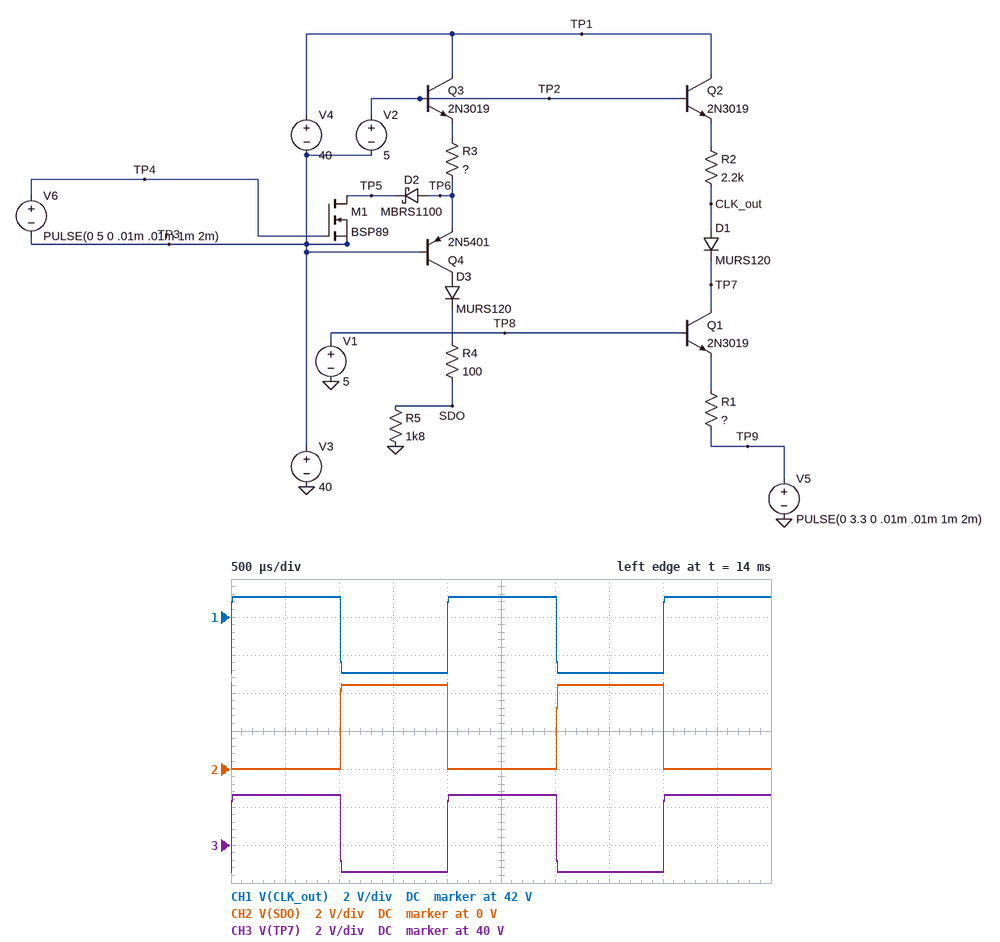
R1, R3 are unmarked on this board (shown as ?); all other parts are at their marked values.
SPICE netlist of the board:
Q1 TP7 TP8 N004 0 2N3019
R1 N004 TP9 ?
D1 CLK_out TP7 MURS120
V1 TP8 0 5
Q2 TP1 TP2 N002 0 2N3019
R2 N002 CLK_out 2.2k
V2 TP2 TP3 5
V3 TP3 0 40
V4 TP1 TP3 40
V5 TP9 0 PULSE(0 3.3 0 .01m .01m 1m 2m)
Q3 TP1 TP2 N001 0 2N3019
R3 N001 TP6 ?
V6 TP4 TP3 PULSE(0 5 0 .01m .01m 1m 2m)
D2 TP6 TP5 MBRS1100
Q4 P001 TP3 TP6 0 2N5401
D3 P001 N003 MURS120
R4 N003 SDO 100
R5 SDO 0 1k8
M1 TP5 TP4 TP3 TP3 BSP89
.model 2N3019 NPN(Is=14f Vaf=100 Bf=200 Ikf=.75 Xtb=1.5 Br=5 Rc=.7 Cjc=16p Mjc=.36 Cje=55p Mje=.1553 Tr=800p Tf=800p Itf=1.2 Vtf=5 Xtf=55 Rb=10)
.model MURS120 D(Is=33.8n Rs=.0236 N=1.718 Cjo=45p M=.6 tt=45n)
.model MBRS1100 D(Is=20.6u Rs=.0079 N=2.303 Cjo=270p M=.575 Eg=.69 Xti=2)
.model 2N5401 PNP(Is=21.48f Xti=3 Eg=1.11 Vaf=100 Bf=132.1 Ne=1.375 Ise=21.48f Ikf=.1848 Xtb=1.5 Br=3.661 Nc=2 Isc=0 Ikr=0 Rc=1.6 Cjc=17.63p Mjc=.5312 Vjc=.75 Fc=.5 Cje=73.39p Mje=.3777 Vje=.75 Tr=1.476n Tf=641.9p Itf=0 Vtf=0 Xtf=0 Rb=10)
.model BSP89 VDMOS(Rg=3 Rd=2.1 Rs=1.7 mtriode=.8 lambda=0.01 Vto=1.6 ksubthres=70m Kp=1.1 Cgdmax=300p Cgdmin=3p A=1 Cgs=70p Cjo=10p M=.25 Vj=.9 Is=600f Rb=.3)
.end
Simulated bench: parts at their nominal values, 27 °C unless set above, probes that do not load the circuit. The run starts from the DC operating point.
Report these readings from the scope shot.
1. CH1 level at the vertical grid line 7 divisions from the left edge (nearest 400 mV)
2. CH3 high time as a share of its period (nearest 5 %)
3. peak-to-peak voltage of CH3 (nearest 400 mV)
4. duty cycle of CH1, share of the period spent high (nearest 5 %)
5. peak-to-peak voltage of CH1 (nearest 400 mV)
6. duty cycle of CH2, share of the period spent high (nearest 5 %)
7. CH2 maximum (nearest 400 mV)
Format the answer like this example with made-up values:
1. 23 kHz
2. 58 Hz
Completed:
1. 39.2 V
2. 50 %
3. 4.0 V
4. 50 %
5. 4.0 V
6. 50 %
7. 4.4 V
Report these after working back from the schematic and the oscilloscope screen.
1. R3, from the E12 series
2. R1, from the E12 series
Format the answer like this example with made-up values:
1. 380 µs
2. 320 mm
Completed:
1. 1.5 kΩ
2. 1.8 kΩ
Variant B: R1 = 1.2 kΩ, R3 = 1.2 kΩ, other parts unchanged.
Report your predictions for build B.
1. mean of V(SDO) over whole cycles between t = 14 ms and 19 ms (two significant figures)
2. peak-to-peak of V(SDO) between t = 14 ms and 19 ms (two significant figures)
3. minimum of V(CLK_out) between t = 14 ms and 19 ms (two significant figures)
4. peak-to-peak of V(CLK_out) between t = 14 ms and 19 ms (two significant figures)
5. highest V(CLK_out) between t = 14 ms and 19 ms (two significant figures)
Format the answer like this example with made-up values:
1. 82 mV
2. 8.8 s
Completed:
1. 2.7 V
2. 5.6 V
3. 36 V
4. 6.0 V
5. 42 V
